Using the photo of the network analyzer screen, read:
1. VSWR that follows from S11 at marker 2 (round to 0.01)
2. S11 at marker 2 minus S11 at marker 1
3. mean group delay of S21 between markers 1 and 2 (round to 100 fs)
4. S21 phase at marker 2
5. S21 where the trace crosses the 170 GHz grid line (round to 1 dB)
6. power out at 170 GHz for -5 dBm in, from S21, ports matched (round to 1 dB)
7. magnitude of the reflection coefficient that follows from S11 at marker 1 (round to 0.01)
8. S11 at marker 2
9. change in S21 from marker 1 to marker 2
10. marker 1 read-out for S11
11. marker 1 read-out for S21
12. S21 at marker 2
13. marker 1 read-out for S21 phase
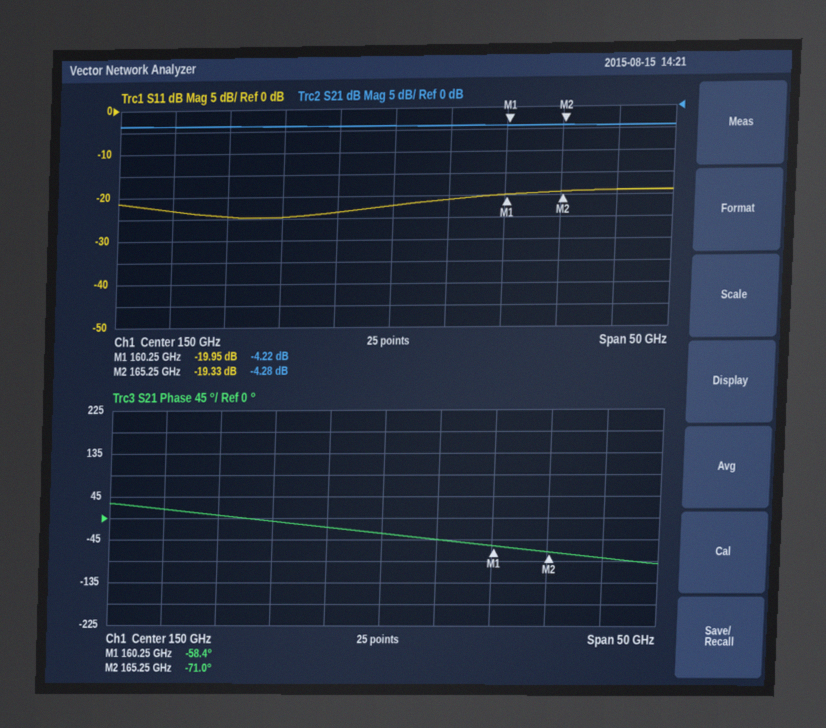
1.24
0.62 dB
7.0 ps
-71.0°
-4 dB
-9 dBm
0.10
-19.33 dB
-0.06 dB
-19.95 dB
-4.22 dB
-4.28 dB
-58.4°
